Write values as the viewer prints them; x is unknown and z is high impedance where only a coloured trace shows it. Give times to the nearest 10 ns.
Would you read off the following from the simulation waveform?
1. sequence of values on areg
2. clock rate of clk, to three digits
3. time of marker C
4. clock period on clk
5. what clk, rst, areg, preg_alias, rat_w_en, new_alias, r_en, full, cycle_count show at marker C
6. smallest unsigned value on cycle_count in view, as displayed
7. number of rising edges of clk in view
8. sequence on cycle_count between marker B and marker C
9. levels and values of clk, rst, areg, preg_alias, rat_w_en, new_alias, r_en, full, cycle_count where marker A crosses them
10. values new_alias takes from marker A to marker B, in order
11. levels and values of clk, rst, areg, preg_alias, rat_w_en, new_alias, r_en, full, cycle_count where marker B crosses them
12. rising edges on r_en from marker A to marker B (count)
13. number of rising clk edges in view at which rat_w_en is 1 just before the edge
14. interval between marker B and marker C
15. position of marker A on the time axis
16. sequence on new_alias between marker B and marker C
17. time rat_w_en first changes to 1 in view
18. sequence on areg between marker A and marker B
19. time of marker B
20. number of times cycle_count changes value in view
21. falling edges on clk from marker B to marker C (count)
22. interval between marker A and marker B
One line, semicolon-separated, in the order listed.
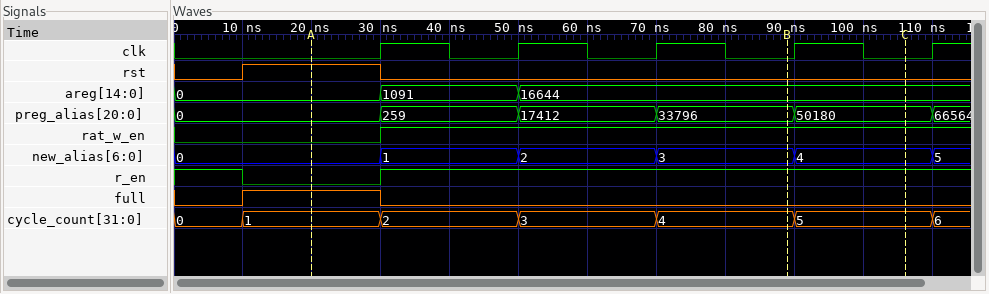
0, 1091, 16644; 50.0 MHz; 110 ns; 20 ns; clk=0, rst=0, areg=16644, preg_alias=50180, rat_w_en=1, new_alias=4, r_en=1, full=0, cycle_count=5; 0; 5; 4, 5; clk=0, rst=1, areg=0, preg_alias=0, rat_w_en=0, new_alias=0, r_en=0, full=1, cycle_count=1; 0, 1, 2, 3; clk=0, rst=0, areg=16644, preg_alias=33796, rat_w_en=1, new_alias=3, r_en=1, full=0, cycle_count=4; 1; 4; 20 ns; 20 ns; 3, 4; 30 ns; 0, 1091, 16644; 90 ns; 6; 1; 70 ns
